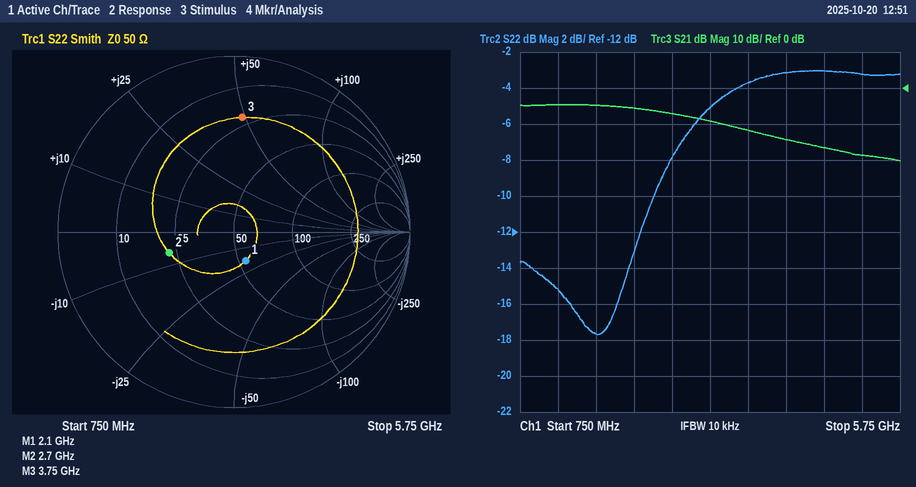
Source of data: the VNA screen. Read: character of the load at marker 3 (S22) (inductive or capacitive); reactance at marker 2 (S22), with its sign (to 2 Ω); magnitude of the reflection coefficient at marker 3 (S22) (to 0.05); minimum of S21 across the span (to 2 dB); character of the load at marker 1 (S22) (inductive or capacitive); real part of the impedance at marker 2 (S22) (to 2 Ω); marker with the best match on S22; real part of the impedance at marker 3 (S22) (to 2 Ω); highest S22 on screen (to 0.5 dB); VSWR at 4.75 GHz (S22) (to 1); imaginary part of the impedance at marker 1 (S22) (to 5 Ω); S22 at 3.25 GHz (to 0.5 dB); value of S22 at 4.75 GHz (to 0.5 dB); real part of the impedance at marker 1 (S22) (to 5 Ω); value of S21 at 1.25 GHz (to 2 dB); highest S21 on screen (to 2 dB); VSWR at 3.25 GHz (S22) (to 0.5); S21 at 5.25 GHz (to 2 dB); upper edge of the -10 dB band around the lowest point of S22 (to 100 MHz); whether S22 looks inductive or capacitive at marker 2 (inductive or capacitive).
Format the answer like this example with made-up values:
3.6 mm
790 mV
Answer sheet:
inductive
-6 Ω
0.65
-20 dB
capacitive
22 Ω
marker 1
22 Ω
-3.0 dB
6
-20 Ω
-5.0 dB
-3.0 dB
55 Ω
-4 dB
-4 dB
3.5
-18 dB
2.5 GHz
capacitive
